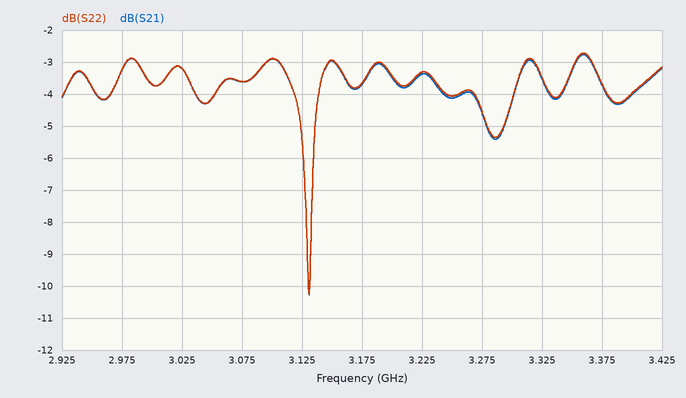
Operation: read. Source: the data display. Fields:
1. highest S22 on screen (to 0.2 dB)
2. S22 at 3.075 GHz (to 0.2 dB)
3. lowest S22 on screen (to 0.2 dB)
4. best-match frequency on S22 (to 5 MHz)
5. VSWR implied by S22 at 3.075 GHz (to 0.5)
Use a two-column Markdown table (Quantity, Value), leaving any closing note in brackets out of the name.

| Quantity | Value |
|---|---|
| highest S22 on screen | -2.8 dB |
| S22 at 3.075 GHz | -3.6 dB |
| lowest S22 on screen | -10.2 dB |
| best-match frequency on S22 | 3.130 GHz |
| VSWR implied by S22 at 3.075 GHz | 5.0 |
